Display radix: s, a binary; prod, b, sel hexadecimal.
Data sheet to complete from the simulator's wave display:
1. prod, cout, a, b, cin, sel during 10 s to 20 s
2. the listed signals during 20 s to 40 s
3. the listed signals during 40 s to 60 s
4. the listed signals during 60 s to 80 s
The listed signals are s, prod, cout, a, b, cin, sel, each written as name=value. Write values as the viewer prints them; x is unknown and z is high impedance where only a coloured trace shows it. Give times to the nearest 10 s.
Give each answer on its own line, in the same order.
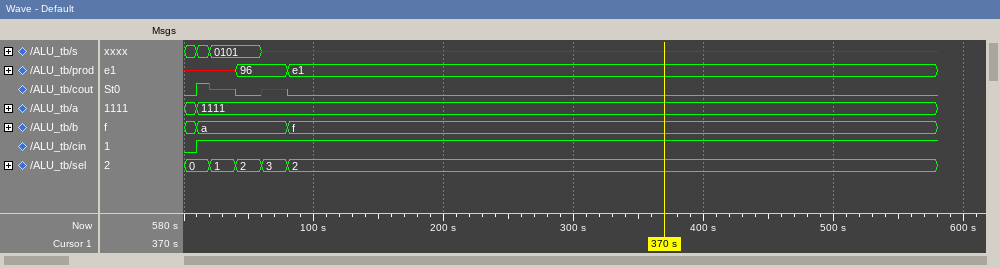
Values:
prod=x, cout=1, a=1111, b=a, cin=1, sel=0
s=0101, prod=x, cout=z, a=1111, b=a, cin=1, sel=1
s=0101, prod=96, cout=0, a=1111, b=a, cin=1, sel=2
s=x, prod=96, cout=x, a=1111, b=a, cin=1, sel=3
